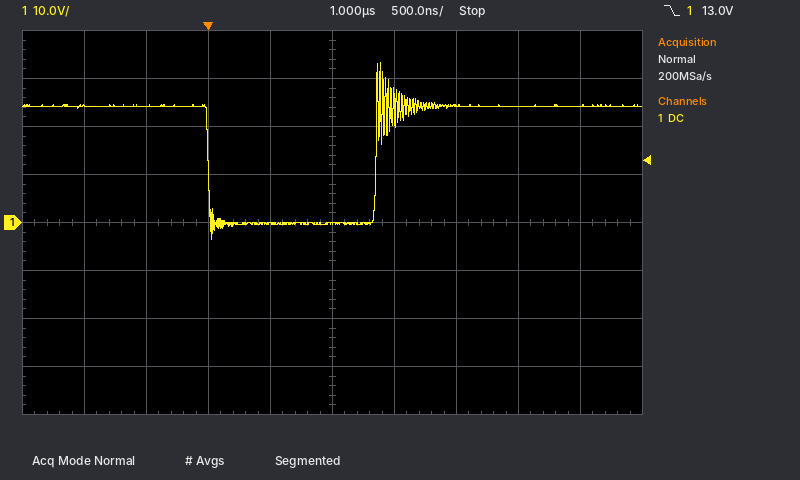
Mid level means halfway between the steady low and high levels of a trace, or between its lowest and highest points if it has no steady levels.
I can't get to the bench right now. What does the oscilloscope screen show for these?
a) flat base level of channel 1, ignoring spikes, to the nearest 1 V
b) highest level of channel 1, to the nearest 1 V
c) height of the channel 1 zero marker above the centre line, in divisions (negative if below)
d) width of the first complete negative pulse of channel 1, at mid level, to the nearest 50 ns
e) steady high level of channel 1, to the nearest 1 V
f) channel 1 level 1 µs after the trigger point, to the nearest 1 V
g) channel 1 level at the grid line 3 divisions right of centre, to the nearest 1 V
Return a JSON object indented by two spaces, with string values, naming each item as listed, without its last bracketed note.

{
  "flat base level of channel 1, ignoring spikes, to the nearest 1 V": "0 V",
  "highest level of channel 1, to the nearest 1 V": "33 V",
  "height of the channel 1 zero marker above the centre line, in divisions": "0.0 div",
  "width of the first complete negative pulse of channel 1, at mid level, to the nearest 50 ns": "1.35 µs",
  "steady high level of channel 1, to the nearest 1 V": "24 V",
  "channel 1 level 1 µs after the trigger point, to the nearest 1 V": "0 V",
  "channel 1 level at the grid line 3 divisions right of centre, to the nearest 1 V": "24 V"
}
